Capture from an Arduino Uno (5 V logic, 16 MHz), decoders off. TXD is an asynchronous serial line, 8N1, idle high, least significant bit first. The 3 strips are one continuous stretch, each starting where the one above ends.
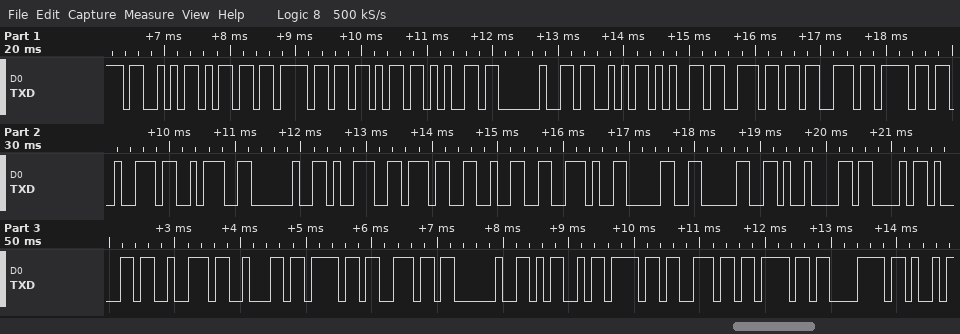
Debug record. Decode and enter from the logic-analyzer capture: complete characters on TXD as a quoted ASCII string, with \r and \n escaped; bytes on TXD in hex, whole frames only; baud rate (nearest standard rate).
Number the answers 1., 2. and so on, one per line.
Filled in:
1. "Smoke Sensor: 972.00\tCarbon Monox"
2. 0x53 0x6D 0x6F 0x6B 0x65 0x20 0x53 0x65 0x6E 0x73 0x6F 0x72 0x3A 0x20 0x39 0x37 0x32 0x2E 0x30 0x30 0x09 0x43 0x61 0x72 0x62 0x6F 0x6E 0x20 0x4D 0x6F 0x6E 0x6F 0x78
3. 9600 baud
